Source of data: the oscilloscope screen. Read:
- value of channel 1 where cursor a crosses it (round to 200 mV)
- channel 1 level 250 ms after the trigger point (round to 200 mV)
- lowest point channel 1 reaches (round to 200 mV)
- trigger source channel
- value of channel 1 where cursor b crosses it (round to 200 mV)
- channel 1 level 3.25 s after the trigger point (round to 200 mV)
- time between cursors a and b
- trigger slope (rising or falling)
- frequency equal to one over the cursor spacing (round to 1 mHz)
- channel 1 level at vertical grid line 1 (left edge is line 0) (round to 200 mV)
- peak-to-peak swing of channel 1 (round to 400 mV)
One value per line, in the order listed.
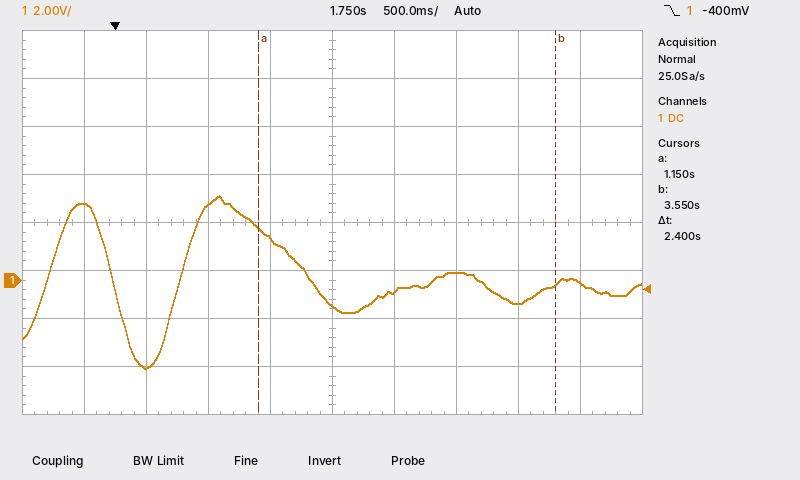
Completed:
2.2 V
-3.6 V
-3.6 V
channel 1
-200 mV
-1.0 V
2.4 s
falling
417 mHz
3.2 V
7.2 V
